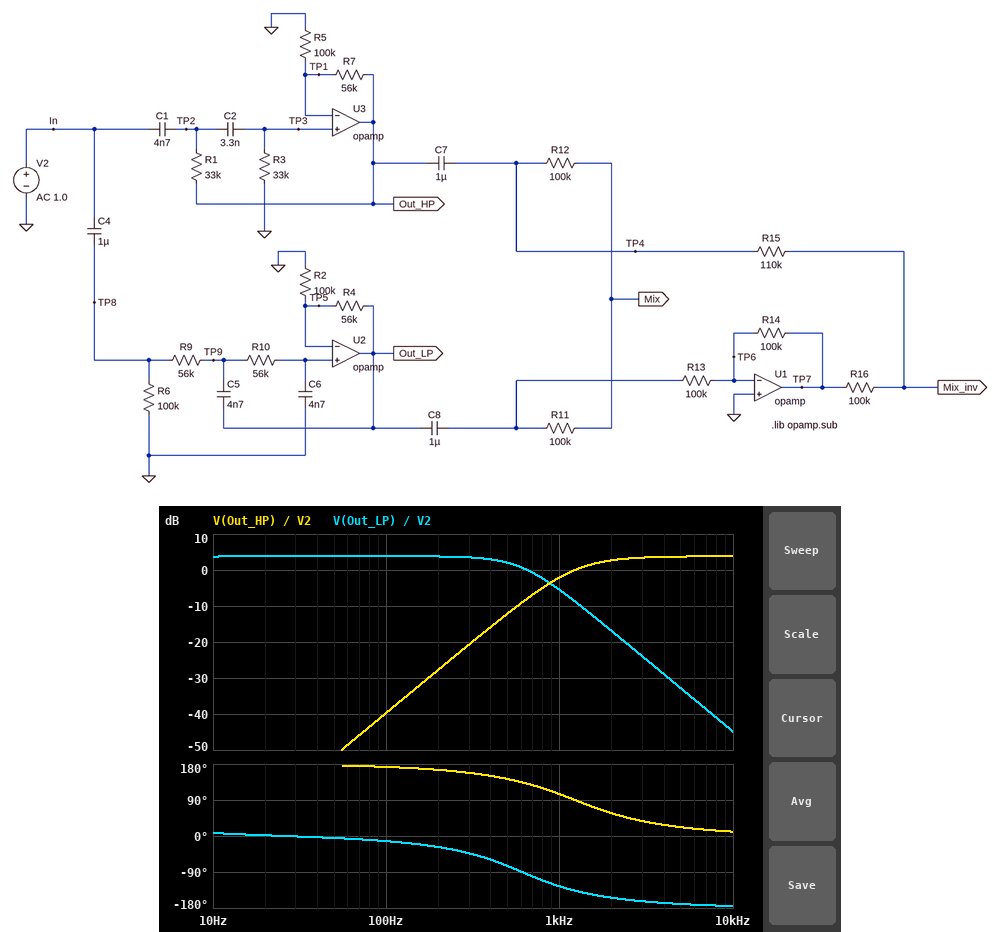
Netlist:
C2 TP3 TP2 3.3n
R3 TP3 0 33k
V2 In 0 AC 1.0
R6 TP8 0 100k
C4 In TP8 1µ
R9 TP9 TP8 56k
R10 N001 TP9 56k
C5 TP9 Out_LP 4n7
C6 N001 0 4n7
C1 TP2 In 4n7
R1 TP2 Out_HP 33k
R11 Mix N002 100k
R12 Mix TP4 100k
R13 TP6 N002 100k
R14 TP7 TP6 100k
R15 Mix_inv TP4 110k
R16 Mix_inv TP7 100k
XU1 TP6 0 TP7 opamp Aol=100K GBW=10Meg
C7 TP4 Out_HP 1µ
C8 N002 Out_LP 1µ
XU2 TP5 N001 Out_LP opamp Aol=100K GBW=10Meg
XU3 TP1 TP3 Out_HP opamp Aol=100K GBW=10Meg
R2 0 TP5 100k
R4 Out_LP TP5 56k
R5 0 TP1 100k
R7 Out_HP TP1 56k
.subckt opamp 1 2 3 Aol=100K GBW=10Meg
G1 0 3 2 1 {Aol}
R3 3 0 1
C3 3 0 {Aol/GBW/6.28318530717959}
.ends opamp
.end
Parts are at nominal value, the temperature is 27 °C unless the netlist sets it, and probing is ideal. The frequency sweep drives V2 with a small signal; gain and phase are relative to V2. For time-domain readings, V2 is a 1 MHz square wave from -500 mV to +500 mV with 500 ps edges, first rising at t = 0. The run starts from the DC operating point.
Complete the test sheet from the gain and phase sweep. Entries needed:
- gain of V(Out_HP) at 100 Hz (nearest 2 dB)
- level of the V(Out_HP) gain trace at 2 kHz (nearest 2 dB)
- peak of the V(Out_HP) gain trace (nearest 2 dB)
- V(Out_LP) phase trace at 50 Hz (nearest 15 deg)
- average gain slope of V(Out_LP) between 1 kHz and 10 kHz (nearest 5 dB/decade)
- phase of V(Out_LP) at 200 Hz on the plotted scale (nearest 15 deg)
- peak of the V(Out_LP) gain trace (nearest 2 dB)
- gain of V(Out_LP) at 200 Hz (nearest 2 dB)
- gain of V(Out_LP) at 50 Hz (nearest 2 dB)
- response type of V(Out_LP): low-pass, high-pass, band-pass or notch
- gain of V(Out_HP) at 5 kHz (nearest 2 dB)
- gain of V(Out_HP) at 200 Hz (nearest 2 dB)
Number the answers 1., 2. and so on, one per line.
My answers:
1. -40 dB
2. 2 dB
3. 4 dB
4. 0 deg
5. -40 dB/decade
6. -30 deg
7. 4 dB
8. 4 dB
9. 4 dB
10. low-pass
11. 4 dB
12. -28 dB
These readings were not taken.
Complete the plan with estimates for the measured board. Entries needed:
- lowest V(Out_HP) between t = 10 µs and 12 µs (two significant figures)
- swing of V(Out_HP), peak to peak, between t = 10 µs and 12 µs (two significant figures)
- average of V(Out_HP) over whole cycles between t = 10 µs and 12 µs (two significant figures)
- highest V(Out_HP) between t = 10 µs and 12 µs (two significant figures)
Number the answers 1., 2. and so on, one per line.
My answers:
1. -110 mV
2. 1.6 V
3. 680 mV
4. 1.5 V
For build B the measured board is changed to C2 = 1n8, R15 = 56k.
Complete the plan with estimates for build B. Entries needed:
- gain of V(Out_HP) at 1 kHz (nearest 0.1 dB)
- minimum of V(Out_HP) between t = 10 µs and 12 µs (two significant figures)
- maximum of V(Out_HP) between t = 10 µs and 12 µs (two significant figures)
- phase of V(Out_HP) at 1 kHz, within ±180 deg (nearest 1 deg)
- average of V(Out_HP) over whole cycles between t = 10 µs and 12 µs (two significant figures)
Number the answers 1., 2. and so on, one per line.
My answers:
1. -7.2 dB
2. -170 mV
3. 1.4 V
4. 119 deg
5. 630 mV
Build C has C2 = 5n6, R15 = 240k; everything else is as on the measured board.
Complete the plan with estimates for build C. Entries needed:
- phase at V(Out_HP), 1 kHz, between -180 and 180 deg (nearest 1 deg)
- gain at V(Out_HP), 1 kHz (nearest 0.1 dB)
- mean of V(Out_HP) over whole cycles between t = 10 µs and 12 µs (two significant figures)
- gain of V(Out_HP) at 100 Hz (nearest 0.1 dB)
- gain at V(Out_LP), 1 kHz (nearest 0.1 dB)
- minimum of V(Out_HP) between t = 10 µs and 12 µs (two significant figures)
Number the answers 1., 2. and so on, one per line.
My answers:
1. 85 deg
2. 1.5 dB
3. 710 mV
4. -35.1 dB
5. -5.5 dB
6. -75 mV
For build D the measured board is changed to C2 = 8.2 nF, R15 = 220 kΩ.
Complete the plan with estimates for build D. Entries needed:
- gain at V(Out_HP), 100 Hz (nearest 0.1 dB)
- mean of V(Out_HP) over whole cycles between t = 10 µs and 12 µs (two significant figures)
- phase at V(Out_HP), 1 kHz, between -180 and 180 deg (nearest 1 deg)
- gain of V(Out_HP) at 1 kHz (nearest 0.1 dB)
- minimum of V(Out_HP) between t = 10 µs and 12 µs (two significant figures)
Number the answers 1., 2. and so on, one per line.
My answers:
1. -31.7 dB
2. 730 mV
3. 69 deg
4. 2.9 dB
5. -60 mV
